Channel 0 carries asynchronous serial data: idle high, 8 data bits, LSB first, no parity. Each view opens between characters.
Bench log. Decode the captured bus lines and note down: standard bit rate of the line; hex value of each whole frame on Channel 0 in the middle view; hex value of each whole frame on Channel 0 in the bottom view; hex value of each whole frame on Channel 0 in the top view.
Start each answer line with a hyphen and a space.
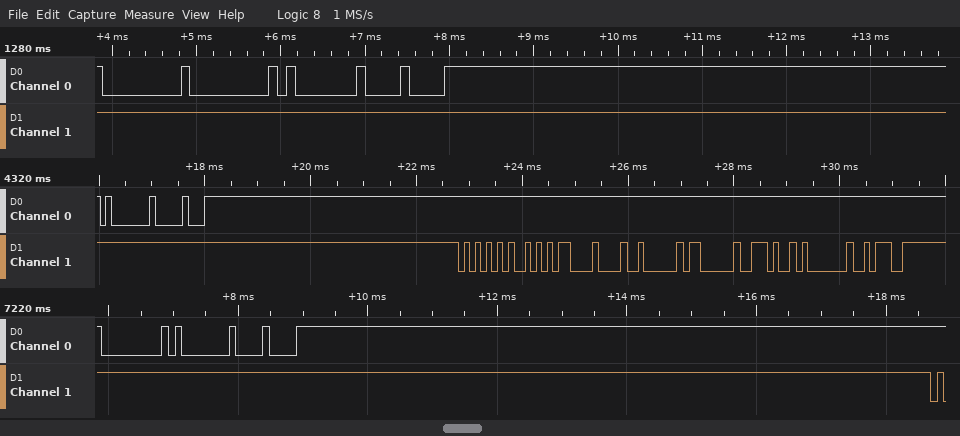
- 9600 baud
- 01, 10
- 00, 01, 08
- 00, 00, 01, 08
